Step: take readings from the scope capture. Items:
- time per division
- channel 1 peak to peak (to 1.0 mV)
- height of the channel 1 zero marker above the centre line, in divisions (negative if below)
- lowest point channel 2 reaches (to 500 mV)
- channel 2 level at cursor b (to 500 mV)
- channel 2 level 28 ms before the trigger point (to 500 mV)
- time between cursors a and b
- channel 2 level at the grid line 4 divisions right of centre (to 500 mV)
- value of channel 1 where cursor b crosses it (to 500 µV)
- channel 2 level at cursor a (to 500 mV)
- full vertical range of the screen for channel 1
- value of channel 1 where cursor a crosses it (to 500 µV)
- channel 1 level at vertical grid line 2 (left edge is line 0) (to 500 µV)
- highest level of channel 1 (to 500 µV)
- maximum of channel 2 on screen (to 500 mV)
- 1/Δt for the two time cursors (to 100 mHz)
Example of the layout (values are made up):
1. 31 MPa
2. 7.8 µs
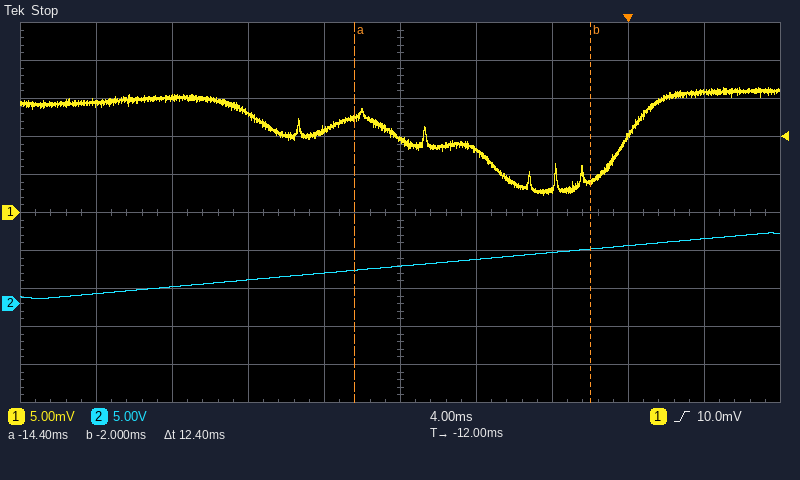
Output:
1. 4 ms
2. 14.0 mV
3. 0.0 div
4. 500 mV
5. 7.0 V
6. 1.5 V
7. 12.4 ms
8. 8.5 V
9. 4.0 mV
10. 4.5 V
11. 50 mV
12. 12.5 mV
13. 15.0 mV
14. 16.5 mV
15. 9.5 V
16. 80.6 Hz
